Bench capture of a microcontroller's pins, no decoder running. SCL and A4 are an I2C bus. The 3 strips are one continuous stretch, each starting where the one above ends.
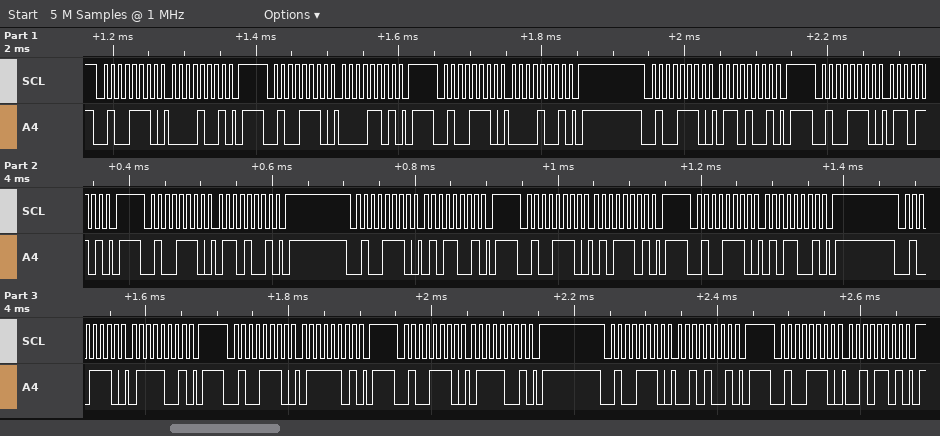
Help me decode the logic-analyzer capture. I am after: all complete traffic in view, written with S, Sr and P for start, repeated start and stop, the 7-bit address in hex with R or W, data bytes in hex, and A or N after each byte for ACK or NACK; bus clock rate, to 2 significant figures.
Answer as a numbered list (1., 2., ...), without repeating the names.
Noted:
1. S 27W A 09 A P S 27W A 0D A P S 27W A 09 A P S 27W A 69 A P S 27W A 6D A P S 27W A 69 A P S 27W A 59 A P S 27W A 5D A P S 27W A 59 A P S 27W A 79 A P S 27W A 7D A P S 27W A 79 A P S 27W A 29 A P S 27W A 2D A P
2. 100 kHz
